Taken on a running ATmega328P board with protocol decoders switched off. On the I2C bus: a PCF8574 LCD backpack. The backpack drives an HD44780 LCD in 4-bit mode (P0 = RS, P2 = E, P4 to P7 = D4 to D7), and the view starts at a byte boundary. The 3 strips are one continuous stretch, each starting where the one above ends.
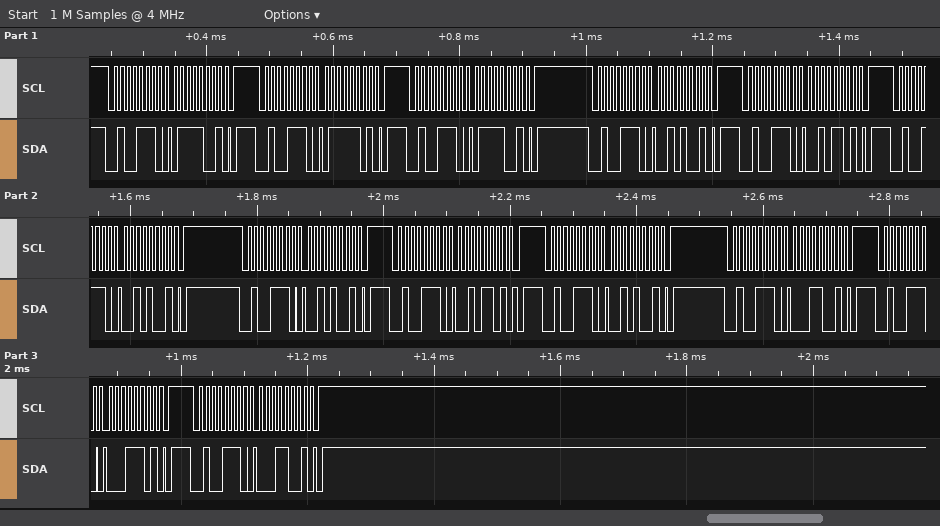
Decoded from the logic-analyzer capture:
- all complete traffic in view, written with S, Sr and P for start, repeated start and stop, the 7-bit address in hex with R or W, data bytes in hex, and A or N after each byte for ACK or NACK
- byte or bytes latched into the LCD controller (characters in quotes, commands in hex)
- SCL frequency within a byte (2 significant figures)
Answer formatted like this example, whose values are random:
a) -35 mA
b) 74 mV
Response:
a) S 27W A 79 A P S 27W A 7D A P S 27W A 79 A P S 27W A 29 A P S 27W A 2D A P S 27W A 29 A P S 27W A 29 A P S 27W A 2D A P S 27W A 29 A P S 27W A 19 A P S 27W A 1D A P S 27W A 19 A P
b) 'r' '!'
c) 100 kHz
